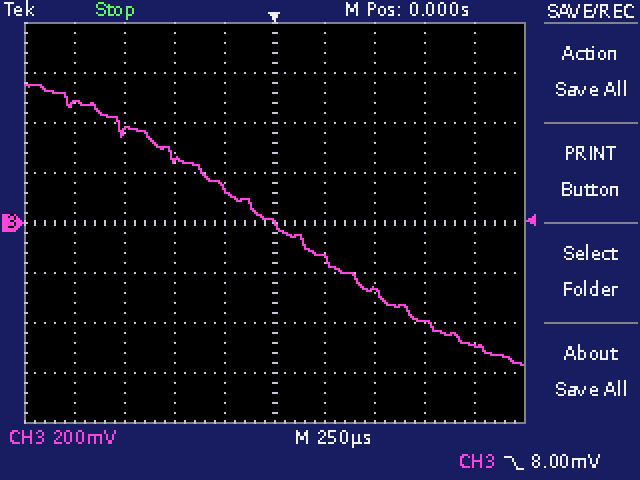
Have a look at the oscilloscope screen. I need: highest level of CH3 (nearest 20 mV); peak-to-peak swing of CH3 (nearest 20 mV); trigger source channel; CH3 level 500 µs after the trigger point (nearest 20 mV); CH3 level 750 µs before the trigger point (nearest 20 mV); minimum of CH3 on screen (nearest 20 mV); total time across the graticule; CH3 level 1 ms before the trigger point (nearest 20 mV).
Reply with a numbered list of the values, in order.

1. 560 mV
2. 1.12 V
3. CH3
4. -260 mV
5. 360 mV
6. -560 mV
7. 2.5 ms
8. 480 mV
